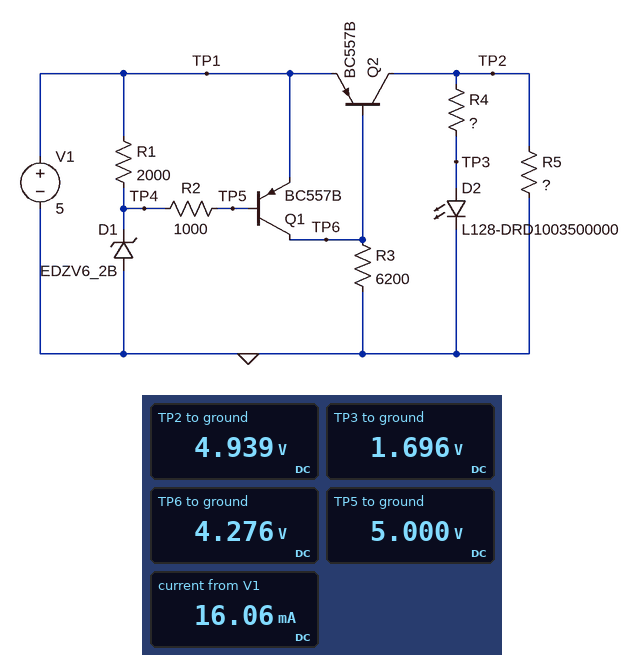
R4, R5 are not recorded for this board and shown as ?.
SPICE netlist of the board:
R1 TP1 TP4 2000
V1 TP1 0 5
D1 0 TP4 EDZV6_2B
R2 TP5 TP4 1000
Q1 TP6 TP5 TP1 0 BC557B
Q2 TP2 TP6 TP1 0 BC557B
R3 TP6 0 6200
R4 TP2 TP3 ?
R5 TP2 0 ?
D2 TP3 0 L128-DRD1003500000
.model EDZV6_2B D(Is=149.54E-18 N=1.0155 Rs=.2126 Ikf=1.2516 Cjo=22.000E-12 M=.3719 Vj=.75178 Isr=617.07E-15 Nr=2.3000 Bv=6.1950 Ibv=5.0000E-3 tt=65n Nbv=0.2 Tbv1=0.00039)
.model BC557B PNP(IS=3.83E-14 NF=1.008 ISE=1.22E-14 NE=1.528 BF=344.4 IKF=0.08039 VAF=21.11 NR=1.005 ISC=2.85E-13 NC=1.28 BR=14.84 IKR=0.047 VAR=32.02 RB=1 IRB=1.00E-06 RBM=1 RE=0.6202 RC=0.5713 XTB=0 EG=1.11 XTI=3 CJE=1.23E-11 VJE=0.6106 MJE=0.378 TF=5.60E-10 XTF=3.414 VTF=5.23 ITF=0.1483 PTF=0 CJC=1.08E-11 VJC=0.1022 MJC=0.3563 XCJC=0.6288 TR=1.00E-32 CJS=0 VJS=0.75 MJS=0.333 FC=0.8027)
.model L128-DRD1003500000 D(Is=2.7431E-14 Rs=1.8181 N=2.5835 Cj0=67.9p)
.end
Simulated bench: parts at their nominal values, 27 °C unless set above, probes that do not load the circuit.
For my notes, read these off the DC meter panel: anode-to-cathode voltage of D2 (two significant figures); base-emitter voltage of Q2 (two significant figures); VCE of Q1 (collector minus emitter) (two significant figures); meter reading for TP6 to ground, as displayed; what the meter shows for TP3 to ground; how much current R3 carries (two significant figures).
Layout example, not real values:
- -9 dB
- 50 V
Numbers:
- 1.7 V
- -720 mV
- -720 mV
- 4.276 V
- 1.696 V
- 690 µA
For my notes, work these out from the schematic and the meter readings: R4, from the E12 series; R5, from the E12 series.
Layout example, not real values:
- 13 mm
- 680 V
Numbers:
- 1.2 kΩ
- 390 Ω
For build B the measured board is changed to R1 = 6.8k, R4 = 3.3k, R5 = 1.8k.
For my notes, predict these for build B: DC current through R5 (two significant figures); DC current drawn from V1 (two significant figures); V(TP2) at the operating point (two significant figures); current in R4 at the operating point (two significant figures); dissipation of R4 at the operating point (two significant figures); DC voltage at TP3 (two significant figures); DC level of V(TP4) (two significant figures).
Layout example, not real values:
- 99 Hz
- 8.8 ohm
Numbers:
- 2.8 mA
- 4.5 mA
- 5.0 V
- 1.0 mA
- 3.4 mW
- 1.6 V
- 5.0 V
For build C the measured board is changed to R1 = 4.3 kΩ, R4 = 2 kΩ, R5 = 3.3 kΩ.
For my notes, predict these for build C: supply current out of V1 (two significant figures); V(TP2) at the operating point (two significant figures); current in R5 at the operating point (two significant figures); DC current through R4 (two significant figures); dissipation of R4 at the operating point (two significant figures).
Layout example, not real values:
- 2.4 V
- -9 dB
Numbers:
- 3.9 mA
- 5.0 V
- 1.5 mA
- 1.7 mA
- 5.5 mW
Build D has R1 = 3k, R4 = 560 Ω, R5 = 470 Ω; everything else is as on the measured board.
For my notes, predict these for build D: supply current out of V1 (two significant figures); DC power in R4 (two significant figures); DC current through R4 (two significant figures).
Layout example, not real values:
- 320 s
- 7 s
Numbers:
- 17 mA
- 18 mW
- 5.7 mA
